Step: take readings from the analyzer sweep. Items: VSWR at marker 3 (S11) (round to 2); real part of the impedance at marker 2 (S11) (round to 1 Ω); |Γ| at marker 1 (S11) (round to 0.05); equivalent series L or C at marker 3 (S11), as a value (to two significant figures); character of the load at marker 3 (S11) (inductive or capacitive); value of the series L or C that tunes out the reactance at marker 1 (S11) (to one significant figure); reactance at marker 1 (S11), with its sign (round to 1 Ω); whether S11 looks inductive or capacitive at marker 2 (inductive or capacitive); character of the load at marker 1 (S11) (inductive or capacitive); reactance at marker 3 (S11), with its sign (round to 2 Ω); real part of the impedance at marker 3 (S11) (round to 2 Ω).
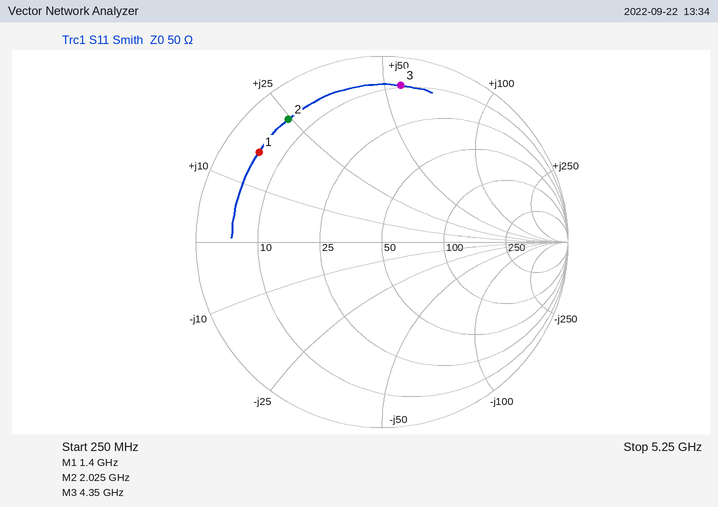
12
6 Ω
0.80
2.0 nH
inductive
7 pF
+16 Ω
inductive
inductive
+56 Ω
10 Ω
